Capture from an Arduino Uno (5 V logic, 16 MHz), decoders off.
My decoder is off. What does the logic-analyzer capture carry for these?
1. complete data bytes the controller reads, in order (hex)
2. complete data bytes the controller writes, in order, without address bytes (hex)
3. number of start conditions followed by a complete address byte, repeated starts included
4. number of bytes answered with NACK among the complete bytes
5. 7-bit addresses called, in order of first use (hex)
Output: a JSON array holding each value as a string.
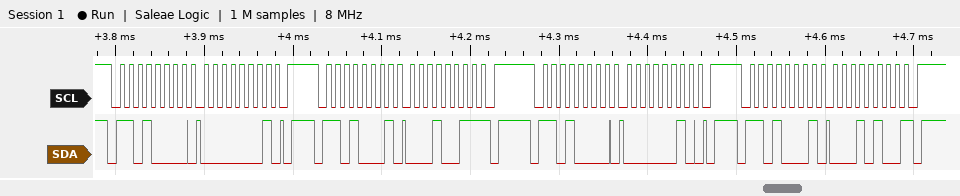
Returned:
["13 14", "01 02", "4", "2", "0x68"]
